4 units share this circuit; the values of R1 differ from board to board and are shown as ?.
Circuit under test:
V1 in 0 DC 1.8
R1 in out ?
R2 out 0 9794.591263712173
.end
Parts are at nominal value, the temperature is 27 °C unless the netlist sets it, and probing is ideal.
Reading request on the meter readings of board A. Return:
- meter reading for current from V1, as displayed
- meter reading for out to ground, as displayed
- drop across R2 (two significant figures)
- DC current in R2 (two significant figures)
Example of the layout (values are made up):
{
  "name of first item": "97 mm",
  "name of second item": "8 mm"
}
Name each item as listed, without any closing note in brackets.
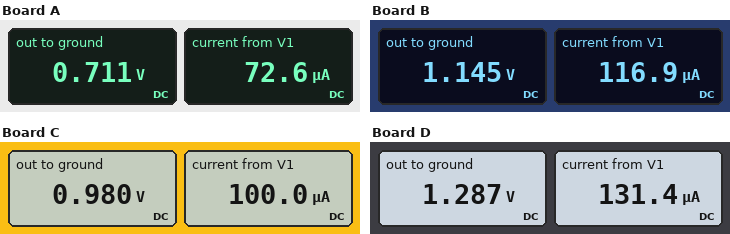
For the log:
{
  "meter reading for current from V1, as displayed": "72.6 µA",
  "meter reading for out to ground, as displayed": "0.711 V",
  "drop across R2": "710 mV",
  "DC current in R2": "73 µA"
}
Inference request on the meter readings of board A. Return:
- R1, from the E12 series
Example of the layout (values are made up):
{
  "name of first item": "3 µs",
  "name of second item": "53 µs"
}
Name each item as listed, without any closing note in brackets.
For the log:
{
  "R1, from the E12 series": "15 kΩ"
}
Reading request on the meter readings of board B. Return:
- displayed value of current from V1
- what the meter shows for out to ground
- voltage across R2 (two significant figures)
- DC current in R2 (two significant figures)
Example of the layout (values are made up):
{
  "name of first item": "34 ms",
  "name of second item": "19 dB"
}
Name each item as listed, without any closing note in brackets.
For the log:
{
  "displayed value of current from V1": "116.9 µA",
  "what the meter shows for out to ground": "1.145 V",
  "voltage across R2": "1.1 V",
  "DC current in R2": "120 µA"
}
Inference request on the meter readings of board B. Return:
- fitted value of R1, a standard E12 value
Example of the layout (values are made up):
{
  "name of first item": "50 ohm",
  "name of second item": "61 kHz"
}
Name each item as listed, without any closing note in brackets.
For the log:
{
  "fitted value of R1, a standard E12 value": "5.6 kΩ"
}
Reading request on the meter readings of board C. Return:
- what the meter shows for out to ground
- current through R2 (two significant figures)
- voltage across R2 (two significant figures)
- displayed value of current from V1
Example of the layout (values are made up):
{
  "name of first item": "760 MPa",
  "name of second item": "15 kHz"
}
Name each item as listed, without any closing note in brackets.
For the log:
{
  "what the meter shows for out to ground": "0.980 V",
  "current through R2": "100 µA",
  "voltage across R2": "980 mV",
  "displayed value of current from V1": "100.0 µA"
}
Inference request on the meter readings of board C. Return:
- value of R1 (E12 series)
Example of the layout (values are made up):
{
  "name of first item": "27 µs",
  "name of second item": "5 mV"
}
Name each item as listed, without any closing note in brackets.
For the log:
{
  "value of R1": "8.2 kΩ"
}
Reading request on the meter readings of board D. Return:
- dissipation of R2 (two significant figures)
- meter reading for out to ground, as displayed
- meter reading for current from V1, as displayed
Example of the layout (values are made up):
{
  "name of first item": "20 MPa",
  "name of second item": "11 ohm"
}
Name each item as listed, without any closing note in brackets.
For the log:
{
  "dissipation of R2": "170 µW",
  "meter reading for out to ground, as displayed": "1.287 V",
  "meter reading for current from V1, as displayed": "131.4 µA"
}
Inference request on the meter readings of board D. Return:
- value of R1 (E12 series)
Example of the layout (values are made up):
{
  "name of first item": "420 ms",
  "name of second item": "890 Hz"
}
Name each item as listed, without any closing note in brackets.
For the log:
{
  "value of R1": "3.9 kΩ"
}
